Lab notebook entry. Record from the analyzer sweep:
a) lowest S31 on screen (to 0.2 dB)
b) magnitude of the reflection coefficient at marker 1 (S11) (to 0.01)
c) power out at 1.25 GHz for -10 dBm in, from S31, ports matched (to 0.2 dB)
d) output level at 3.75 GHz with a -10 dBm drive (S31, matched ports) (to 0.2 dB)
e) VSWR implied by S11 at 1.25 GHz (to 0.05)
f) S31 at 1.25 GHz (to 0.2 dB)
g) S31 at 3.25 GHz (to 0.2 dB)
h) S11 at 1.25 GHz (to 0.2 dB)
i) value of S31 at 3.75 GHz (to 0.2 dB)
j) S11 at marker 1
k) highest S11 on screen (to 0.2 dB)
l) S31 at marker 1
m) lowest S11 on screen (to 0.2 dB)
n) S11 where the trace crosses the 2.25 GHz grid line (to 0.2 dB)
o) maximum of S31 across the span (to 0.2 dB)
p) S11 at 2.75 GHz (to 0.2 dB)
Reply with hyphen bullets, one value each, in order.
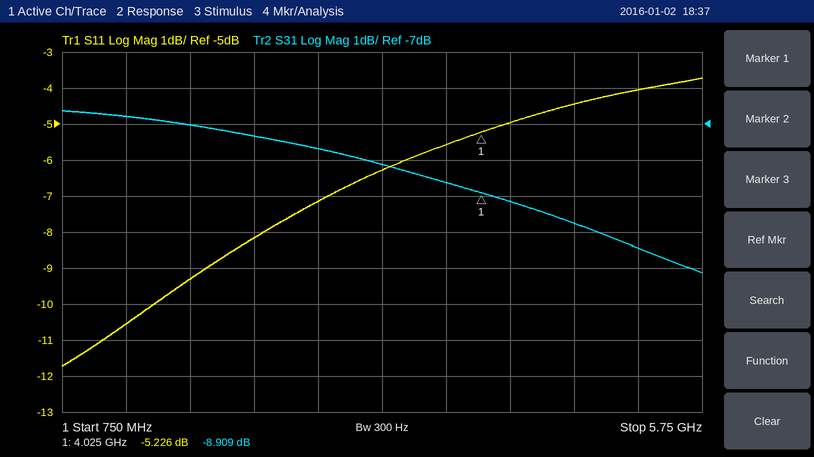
- -11.2 dB
- 0.55
- -16.8 dBm
- -18.6 dBm
- 1.85
- -6.8 dB
- -8.2 dB
- -10.6 dB
- -8.6 dB
- -5.226 dB
- -3.8 dB
- -8.909 dB
- -11.8 dB
- -8.2 dB
- -6.6 dB
- -7.2 dB
